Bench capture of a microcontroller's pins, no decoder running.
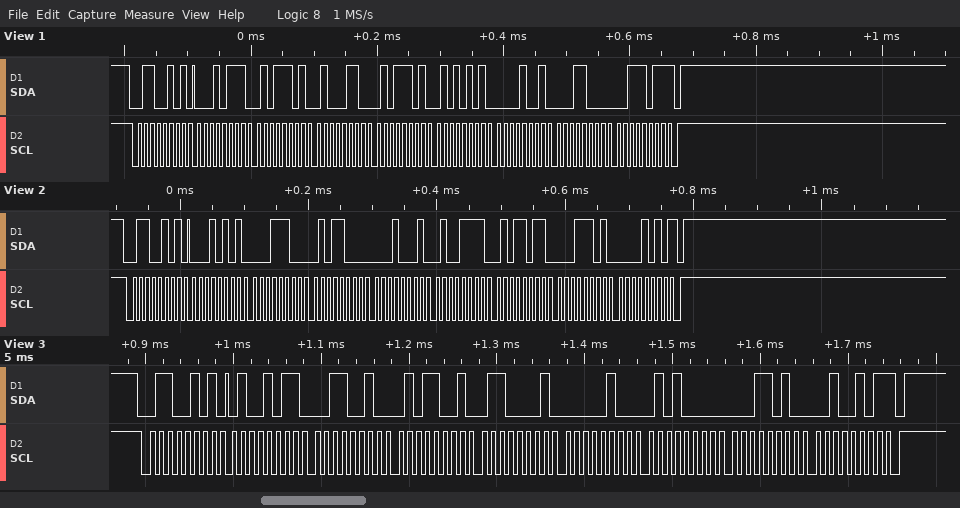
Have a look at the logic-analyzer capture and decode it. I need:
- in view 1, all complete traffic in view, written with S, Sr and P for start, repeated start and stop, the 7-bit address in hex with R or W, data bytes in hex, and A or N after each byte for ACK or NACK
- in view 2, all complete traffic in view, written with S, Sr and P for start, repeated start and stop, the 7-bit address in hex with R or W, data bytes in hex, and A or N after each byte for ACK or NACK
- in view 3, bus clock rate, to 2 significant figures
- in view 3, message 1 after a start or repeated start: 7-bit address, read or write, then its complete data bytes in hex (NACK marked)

S 32R A 17 A 5D A 46 A 5D A 55 A 09 A 18 A 3B N P
S 32R A 15 A 1C A 58 A 11 A 4F A 5B A 1D A 0A N P
100 kHz
0x32 read: 4B 32 59 61 04 50 1A 25 NACK
